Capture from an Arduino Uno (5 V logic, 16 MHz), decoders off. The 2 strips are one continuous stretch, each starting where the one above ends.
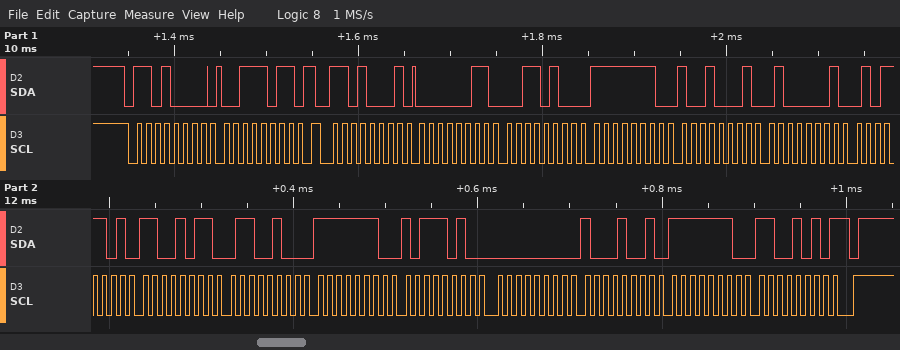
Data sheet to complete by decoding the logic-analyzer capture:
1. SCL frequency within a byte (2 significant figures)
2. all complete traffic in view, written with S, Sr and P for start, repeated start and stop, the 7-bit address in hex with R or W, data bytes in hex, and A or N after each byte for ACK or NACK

100 kHz
S 68W A 3B A Sr 68R A 03 A 34 A FE A 91 A 41 A 5D A CB A 64 A FE A BA A 00 A 89 A FE A CA N P
